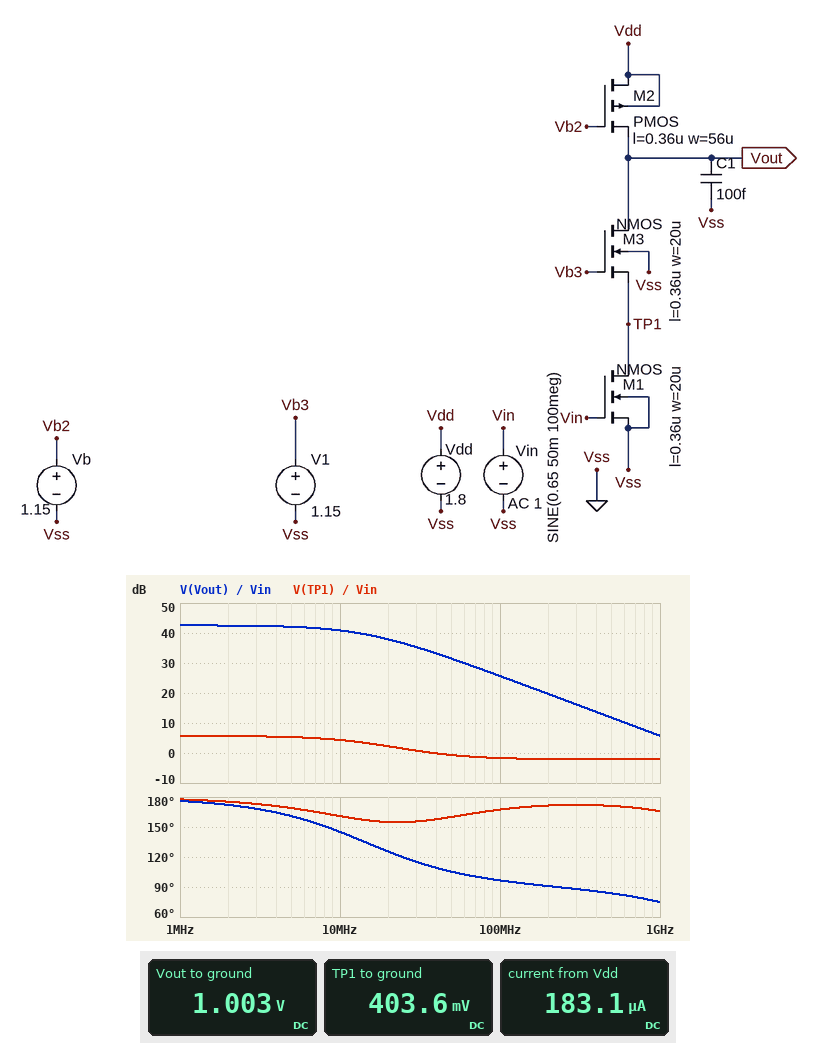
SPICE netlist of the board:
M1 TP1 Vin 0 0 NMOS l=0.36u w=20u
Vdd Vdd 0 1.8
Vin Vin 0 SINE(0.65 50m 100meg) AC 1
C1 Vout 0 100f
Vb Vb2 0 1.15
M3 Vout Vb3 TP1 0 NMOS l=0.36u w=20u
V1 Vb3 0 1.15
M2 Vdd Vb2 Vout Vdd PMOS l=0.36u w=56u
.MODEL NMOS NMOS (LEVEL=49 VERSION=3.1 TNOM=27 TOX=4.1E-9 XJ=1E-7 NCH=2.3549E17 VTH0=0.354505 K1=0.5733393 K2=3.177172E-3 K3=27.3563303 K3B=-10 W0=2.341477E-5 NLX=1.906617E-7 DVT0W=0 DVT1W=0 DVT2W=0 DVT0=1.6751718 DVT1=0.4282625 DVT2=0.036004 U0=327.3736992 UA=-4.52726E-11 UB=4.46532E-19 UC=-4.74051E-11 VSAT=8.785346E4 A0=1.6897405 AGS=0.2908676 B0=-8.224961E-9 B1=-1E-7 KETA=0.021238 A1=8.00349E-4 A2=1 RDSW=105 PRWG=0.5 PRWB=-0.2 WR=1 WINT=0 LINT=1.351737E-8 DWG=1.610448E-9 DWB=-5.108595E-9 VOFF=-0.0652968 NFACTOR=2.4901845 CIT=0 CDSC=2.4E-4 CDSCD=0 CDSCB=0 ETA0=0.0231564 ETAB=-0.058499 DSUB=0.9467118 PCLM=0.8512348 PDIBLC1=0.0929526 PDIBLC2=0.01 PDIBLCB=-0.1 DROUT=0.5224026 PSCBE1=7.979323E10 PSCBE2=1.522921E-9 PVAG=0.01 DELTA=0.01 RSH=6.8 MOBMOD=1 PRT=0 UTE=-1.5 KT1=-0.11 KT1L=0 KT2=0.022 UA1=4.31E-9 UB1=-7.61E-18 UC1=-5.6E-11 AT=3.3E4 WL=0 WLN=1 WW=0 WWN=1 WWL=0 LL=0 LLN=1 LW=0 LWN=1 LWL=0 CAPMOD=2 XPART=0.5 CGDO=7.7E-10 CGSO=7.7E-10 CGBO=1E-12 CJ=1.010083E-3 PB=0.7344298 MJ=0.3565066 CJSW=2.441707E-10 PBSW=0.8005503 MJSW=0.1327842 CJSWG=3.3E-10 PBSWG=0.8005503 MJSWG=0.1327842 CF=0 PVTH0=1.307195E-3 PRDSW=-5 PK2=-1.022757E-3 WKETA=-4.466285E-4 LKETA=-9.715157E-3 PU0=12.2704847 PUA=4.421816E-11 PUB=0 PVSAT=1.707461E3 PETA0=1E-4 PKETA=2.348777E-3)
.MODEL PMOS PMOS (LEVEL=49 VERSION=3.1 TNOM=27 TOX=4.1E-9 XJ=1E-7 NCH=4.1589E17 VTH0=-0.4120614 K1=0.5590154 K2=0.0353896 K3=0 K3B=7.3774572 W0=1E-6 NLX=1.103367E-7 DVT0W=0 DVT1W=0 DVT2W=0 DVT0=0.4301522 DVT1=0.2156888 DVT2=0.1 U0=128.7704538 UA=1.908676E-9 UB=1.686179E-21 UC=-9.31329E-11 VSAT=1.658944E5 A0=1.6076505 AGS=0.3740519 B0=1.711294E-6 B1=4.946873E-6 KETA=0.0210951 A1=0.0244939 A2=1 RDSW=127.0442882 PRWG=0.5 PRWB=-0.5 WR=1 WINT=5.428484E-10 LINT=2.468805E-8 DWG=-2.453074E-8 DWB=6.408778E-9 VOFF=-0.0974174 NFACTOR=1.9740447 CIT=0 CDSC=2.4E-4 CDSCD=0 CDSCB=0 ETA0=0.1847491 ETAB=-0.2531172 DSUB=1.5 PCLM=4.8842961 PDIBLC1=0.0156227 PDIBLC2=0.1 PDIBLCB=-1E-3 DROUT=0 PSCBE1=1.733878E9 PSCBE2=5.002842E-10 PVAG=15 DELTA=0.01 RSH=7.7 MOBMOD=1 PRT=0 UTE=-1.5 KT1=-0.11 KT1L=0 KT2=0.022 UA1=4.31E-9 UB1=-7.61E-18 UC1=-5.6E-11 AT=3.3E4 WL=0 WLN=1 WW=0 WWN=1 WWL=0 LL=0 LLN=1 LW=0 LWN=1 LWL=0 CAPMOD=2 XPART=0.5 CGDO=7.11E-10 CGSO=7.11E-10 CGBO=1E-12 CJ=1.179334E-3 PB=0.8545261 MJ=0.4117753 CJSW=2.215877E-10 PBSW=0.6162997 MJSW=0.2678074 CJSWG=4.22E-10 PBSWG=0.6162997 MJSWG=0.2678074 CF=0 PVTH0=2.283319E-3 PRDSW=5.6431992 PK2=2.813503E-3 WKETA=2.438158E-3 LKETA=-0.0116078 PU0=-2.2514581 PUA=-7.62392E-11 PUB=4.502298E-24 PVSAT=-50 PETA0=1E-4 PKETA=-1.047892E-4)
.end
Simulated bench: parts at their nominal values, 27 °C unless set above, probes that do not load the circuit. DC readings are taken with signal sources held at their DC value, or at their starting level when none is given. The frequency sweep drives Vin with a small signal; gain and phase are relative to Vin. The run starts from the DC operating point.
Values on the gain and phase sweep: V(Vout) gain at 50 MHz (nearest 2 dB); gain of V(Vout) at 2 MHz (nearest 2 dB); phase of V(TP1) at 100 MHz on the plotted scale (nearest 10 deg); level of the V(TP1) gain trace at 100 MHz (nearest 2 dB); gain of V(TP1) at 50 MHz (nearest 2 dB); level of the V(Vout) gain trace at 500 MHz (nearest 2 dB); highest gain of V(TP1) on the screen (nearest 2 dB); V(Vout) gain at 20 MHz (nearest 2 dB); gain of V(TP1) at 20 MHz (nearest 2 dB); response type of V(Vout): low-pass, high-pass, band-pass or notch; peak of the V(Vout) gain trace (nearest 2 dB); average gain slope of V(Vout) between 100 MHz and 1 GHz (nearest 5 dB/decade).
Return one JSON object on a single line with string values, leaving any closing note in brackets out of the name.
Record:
{"V(Vout) gain at 50 MHz": "32 dB", "gain of V(Vout) at 2 MHz": "42 dB", "phase of V(TP1) at 100 MHz on the plotted scale": "170 deg", "level of the V(TP1) gain trace at 100 MHz": "-2 dB", "gain of V(TP1) at 50 MHz": "0 dB", "level of the V(Vout) gain trace at 500 MHz": "12 dB", "highest gain of V(TP1) on the screen": "6 dB", "V(Vout) gain at 20 MHz": "38 dB", "gain of V(TP1) at 20 MHz": "2 dB", "response type of V(Vout): low-pass, high-pass, band-pass or notch": "low-pass", "peak of the V(Vout) gain trace": "42 dB", "average gain slope of V(Vout) between 100 MHz and 1 GHz": "-20 dB/decade"}
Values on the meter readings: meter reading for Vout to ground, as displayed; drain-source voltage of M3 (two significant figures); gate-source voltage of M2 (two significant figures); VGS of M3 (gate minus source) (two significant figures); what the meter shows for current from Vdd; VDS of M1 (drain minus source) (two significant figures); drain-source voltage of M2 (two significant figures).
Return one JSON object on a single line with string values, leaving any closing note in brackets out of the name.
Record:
{"meter reading for Vout to ground, as displayed": "1.003 V", "drain-source voltage of M3": "600 mV", "gate-source voltage of M2": "150 mV", "VGS of M3 (gate minus source)": "750 mV", "what the meter shows for current from Vdd": "183.1 µA", "VDS of M1 (drain minus source)": "400 mV", "drain-source voltage of M2": "800 mV"}
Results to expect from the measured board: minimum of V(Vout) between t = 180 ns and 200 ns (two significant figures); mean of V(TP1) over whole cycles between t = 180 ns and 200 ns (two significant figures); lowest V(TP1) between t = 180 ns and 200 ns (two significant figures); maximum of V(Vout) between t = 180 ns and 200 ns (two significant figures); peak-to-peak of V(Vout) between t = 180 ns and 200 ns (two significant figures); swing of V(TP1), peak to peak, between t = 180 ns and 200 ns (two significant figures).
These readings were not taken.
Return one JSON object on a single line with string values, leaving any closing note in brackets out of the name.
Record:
{"minimum of V(Vout) between t = 180 ns and 200 ns": "140 mV", "mean of V(TP1) over whole cycles between t = 180 ns and 200 ns": "330 mV", "lowest V(TP1) between t = 180 ns and 200 ns": "110 mV", "maximum of V(Vout) between t = 180 ns and 200 ns": "1.7 V", "peak-to-peak of V(Vout) between t = 180 ns and 200 ns": "1.5 V", "swing of V(TP1), peak to peak, between t = 180 ns and 200 ns": "330 mV"}
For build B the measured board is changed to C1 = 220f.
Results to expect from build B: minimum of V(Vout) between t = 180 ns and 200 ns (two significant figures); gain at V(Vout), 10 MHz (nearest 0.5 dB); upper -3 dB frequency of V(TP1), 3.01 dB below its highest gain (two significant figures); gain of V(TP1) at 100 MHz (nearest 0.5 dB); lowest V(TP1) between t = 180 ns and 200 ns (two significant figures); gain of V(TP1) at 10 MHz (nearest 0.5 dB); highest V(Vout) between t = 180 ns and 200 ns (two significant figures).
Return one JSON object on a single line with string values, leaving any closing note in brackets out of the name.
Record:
{"minimum of V(Vout) between t = 180 ns and 200 ns": "200 mV", "gain at V(Vout), 10 MHz": "39.0 dB", "upper -3 dB frequency of V(TP1), 3.01 dB below its highest gain": "11 MHz", "gain of V(TP1) at 100 MHz": "-2.0 dB", "lowest V(TP1) between t = 180 ns and 200 ns": "160 mV", "gain of V(TP1) at 10 MHz": "3.0 dB", "highest V(Vout) between t = 180 ns and 200 ns": "1.2 V"}
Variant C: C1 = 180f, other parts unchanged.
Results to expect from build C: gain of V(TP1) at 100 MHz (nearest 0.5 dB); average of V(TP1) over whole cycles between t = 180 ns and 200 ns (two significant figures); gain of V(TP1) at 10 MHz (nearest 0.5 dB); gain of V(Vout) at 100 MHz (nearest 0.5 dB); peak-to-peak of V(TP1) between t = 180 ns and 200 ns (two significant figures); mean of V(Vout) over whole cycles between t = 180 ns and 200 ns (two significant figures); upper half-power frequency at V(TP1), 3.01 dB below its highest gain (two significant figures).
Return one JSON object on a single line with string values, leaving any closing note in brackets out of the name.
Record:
{"gain of V(TP1) at 100 MHz": "-2.0 dB", "average of V(TP1) over whole cycles between t = 180 ns and 200 ns": "340 mV", "gain of V(TP1) at 10 MHz": "3.5 dB", "gain of V(Vout) at 100 MHz": "22.5 dB", "peak-to-peak of V(TP1) between t = 180 ns and 200 ns": "290 mV", "mean of V(Vout) over whole cycles between t = 180 ns and 200 ns": "740 mV", "upper half-power frequency at V(TP1), 3.01 dB below its highest gain": "12 MHz"}
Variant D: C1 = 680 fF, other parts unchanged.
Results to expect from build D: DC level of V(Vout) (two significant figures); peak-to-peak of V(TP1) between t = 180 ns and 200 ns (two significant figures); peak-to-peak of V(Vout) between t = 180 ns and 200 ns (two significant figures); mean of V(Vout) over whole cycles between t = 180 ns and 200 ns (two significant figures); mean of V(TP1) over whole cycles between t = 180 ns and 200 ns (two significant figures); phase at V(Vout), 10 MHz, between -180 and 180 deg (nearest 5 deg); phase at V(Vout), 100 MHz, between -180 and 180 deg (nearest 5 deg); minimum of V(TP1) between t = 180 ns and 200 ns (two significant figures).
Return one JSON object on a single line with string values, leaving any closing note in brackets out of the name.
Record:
{"DC level of V(Vout)": "1.0 V", "peak-to-peak of V(TP1) between t = 180 ns and 200 ns": "150 mV", "peak-to-peak of V(Vout) between t = 180 ns and 200 ns": "440 mV", "mean of V(Vout) over whole cycles between t = 180 ns and 200 ns": "550 mV", "mean of V(TP1) over whole cycles between t = 180 ns and 200 ns": "370 mV", "phase at V(Vout), 10 MHz, between -180 and 180 deg": "110 deg", "phase at V(Vout), 100 MHz, between -180 and 180 deg": "90 deg", "minimum of V(TP1) between t = 180 ns and 200 ns": "290 mV"}
